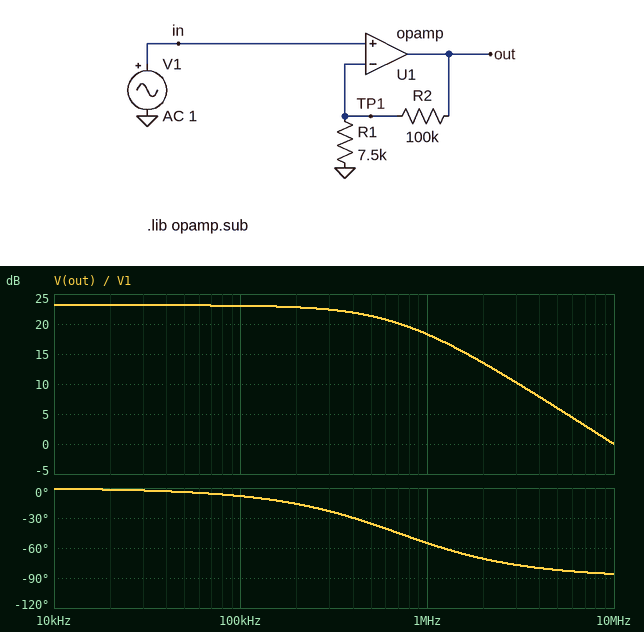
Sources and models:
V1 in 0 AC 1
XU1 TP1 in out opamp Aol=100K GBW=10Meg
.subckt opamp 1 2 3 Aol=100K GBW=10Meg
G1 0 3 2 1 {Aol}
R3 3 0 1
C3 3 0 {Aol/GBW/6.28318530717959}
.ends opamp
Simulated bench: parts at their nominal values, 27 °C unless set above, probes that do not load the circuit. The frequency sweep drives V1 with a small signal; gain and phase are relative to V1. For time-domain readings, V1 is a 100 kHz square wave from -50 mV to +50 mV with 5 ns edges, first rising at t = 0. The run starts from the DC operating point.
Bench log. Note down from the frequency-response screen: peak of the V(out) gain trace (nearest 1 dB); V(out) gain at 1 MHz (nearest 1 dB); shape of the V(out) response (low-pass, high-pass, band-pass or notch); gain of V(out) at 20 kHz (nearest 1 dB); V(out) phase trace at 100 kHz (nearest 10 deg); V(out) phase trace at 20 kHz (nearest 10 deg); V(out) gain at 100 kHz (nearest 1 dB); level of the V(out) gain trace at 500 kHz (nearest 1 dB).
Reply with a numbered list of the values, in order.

1. 23 dB
2. 18 dB
3. low-pass
4. 23 dB
5. -10 deg
6. 0 deg
7. 23 dB
8. 21 dB
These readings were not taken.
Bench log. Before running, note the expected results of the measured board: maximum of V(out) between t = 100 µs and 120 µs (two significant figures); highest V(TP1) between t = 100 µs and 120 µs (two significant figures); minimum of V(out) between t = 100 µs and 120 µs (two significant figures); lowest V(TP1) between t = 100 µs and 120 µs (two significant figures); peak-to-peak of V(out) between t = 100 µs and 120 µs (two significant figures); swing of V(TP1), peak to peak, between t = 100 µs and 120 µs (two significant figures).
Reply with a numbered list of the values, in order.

1. 720 mV
2. 50 mV
3. -720 mV
4. -50 mV
5. 1.4 V
6. 100 mV
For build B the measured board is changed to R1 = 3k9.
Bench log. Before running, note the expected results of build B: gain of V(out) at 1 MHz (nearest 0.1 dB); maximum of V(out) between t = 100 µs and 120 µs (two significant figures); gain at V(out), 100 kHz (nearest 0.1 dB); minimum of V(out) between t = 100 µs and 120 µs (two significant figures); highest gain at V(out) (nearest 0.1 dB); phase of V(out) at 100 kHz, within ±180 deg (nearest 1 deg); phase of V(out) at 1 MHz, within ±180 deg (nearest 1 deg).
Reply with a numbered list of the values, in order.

1. 19.4 dB
2. 1.3 V
3. 28.2 dB
4. -1.3 V
5. 28.5 dB
6. -15 deg
7. -69 deg
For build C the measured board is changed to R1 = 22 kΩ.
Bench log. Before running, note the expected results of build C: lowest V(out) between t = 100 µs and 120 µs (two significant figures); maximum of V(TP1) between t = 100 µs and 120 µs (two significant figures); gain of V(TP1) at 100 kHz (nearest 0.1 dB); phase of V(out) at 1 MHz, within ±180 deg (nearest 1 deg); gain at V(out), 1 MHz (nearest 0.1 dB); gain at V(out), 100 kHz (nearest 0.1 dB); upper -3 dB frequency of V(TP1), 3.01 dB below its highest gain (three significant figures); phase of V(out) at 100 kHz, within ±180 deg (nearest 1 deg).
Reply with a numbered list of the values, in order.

1. -280 mV
2. 50 mV
3. 0 dB
4. -29 deg
5. 13.7 dB
6. 14.9 dB
7. 1.80 MHz
8. -3 deg
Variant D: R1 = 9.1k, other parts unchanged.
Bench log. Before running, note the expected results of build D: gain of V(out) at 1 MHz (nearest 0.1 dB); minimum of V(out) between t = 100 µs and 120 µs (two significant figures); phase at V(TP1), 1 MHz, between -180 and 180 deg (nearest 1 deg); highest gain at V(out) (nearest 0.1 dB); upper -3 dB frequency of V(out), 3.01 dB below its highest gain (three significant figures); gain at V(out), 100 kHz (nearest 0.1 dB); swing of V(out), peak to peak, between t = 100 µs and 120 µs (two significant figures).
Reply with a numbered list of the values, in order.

1. 17.7 dB
2. -600 mV
3. -50 deg
4. 21.6 dB
5. 834 kHz
6. 21.5 dB
7. 1.2 V
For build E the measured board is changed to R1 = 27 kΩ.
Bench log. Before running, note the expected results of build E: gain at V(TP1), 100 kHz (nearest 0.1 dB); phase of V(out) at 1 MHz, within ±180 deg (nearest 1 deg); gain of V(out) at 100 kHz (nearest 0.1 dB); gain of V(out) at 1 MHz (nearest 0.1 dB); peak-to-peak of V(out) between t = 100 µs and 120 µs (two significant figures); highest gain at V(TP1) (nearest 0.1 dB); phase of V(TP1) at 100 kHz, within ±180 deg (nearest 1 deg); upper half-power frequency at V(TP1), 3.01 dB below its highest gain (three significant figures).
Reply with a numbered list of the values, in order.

1. 0 dB
2. -25 deg
3. 13.4 dB
4. 12.6 dB
5. 470 mV
6. 0 dB
7. -3 deg
8. 2.13 MHz
